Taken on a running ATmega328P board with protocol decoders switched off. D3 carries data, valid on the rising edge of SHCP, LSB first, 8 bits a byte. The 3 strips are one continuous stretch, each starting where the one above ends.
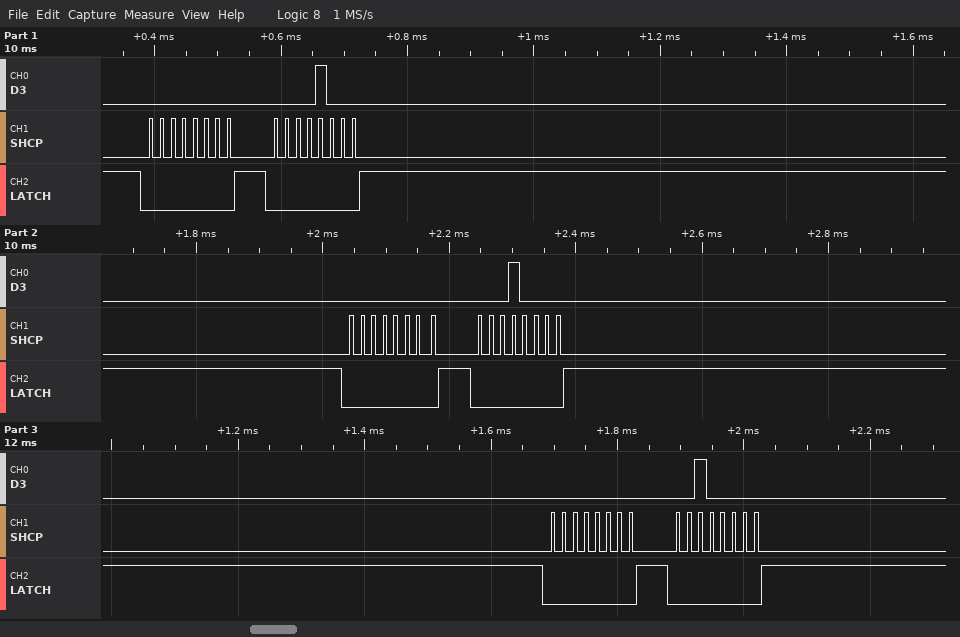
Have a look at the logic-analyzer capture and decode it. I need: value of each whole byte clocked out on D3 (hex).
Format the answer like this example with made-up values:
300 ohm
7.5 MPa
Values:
00 10 00 08 00 04
